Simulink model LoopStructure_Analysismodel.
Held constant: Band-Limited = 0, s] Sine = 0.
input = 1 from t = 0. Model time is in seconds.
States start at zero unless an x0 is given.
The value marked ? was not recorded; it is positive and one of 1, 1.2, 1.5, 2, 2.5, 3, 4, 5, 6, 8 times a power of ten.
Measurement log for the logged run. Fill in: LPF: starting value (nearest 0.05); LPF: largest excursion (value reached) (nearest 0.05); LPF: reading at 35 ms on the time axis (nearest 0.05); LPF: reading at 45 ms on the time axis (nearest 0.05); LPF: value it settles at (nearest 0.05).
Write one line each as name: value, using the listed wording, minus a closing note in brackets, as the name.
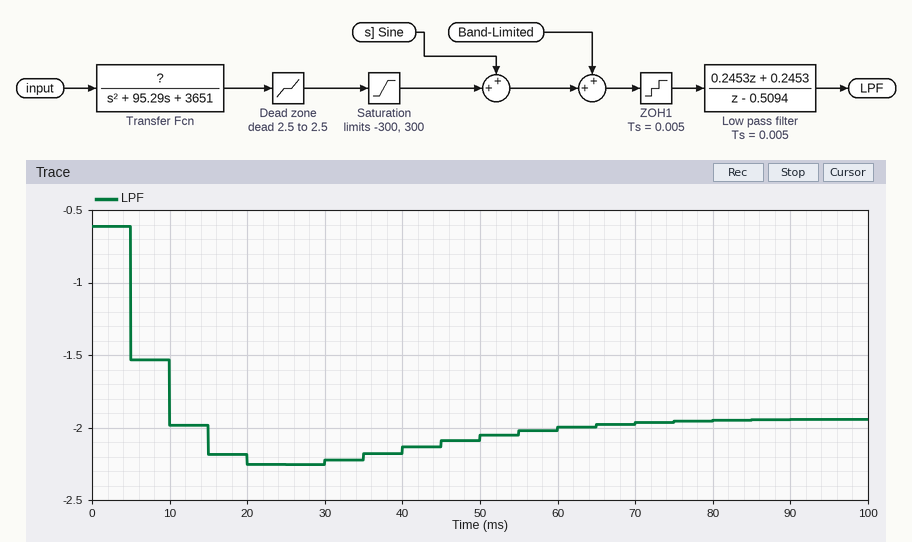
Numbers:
LPF: starting value: -0.60
LPF: largest excursion (value reached): -2.25
LPF: reading at 35 ms on the time axis: -2.20
LPF: reading at 45 ms on the time axis: -2.10
LPF: value it settles at: -1.95
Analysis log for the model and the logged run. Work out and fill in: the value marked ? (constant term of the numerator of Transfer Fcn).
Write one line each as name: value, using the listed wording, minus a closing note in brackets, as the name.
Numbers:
the value marked ?: 2000
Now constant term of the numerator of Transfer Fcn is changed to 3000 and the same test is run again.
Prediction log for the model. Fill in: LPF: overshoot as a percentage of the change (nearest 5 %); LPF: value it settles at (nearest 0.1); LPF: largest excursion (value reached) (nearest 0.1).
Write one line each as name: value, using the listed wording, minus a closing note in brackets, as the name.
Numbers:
LPF: overshoot as a percentage of the change: 50 %
LPF: value it settles at: -1.7
LPF: largest excursion (value reached): -2.2
